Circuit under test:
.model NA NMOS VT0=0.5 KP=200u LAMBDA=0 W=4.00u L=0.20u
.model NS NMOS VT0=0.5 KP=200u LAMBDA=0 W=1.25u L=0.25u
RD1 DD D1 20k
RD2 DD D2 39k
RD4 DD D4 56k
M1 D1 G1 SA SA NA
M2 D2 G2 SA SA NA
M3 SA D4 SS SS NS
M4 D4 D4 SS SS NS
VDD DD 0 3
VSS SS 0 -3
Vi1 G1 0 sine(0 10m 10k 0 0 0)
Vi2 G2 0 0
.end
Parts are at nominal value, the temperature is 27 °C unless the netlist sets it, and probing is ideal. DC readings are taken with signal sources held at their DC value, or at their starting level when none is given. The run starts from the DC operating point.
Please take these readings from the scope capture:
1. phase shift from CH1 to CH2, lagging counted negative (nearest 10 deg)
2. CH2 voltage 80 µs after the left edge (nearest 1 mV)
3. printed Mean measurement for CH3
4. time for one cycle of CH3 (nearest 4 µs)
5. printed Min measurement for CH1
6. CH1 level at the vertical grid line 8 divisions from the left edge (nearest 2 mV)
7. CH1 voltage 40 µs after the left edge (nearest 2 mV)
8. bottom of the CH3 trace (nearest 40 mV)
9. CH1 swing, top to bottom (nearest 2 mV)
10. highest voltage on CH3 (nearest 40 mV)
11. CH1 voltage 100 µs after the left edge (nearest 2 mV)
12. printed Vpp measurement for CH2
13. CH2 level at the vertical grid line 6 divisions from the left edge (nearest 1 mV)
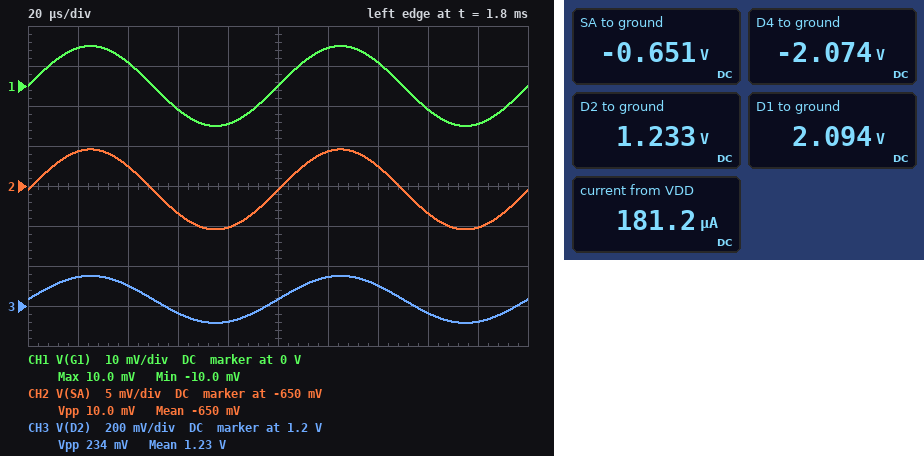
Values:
0 deg
-655 mV
1.23 V
100 µs
-10.0 mV
-6 mV
6 mV
1.12 V
20 mV
1.36 V
0 V
10.0 mV
-646 mV
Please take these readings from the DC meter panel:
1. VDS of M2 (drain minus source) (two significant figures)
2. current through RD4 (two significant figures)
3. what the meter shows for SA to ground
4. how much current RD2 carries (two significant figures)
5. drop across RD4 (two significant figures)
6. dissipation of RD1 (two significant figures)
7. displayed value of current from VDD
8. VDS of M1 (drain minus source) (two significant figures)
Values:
1.9 V
91 µA
-0.651 V
45 µA
5.1 V
41 µW
181.2 µA
2.7 V
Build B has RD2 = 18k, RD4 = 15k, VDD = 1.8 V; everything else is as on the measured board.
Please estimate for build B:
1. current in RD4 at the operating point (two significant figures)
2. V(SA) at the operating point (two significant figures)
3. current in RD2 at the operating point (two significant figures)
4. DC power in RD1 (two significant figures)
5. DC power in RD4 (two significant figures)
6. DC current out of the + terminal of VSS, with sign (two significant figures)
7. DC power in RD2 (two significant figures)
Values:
240 µA
-750 mV
120 µA
280 µW
870 µW
-480 µA
270 µW
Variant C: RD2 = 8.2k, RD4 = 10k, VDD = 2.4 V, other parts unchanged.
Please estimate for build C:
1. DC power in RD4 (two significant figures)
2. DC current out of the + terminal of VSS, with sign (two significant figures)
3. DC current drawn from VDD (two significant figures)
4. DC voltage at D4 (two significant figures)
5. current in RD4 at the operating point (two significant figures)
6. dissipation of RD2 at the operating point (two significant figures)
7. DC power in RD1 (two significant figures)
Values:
1.6 mW
-800 µA
800 µA
-1.6 V
400 µA
490 µW
480 µW
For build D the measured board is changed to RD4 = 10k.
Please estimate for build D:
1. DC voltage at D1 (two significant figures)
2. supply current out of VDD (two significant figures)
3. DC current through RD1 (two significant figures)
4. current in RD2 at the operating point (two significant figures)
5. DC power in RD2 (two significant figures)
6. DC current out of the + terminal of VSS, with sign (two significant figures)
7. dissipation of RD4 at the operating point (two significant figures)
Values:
-2.3 V
860 µA
270 µA
140 µA
730 µW
-860 µA
2.1 mW
